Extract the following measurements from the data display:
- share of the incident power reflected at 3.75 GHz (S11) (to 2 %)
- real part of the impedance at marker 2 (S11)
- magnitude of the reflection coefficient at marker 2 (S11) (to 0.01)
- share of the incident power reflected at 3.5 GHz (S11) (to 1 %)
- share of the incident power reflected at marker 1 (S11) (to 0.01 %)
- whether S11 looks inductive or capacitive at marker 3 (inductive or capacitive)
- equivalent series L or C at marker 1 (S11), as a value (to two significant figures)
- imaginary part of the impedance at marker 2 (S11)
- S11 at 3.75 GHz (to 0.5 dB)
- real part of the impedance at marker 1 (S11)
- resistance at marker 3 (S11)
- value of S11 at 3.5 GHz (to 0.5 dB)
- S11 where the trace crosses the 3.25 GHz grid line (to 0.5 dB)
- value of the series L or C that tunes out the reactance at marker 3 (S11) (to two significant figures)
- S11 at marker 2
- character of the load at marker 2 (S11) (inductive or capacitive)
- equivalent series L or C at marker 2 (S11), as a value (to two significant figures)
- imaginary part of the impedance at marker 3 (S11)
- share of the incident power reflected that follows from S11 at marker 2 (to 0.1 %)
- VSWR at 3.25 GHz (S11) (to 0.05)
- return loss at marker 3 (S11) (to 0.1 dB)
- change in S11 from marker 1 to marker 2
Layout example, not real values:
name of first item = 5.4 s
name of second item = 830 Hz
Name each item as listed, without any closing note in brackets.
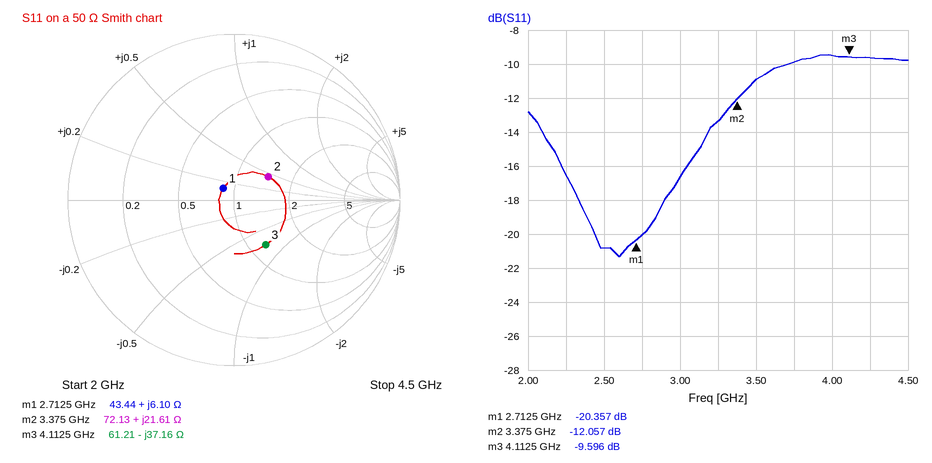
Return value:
share of the incident power reflected at 3.75 GHz (S11) = 10 %
real part of the impedance at marker 2 = 72.13 Ω
magnitude of the reflection coefficient at marker 2 (S11) = 0.25
share of the incident power reflected at 3.5 GHz (S11) = 8 %
share of the incident power reflected at marker 1 (S11) = 0.92 %
whether S11 looks inductive or capacitive at marker 3 = capacitive
equivalent series L or C at marker 1 (S11), as a value = 360 pH
imaginary part of the impedance at marker 2 = +21.61 Ω
S11 at 3.75 GHz = -10.0 dB
real part of the impedance at marker 1 = 43.44 Ω
resistance at marker 3 = 61.21 Ω
value of S11 at 3.5 GHz = -11.0 dB
S11 where the trace crosses the 3.25 GHz grid line = -13.5 dB
value of the series L or C that tunes out the reactance at marker 3 (S11) = 1.4 nH
S11 at marker 2 = -12.057 dB
character of the load at marker 2 (S11) = inductive
equivalent series L or C at marker 2 (S11), as a value = 1.0 nH
imaginary part of the impedance at marker 3 = -37.16 Ω
share of the incident power reflected that follows from S11 at marker 2 = 6.2 %
VSWR at 3.25 GHz (S11) = 1.55
return loss at marker 3 (S11) = 9.6 dB
change in S11 from marker 1 to marker 2 = 8.300 dB
